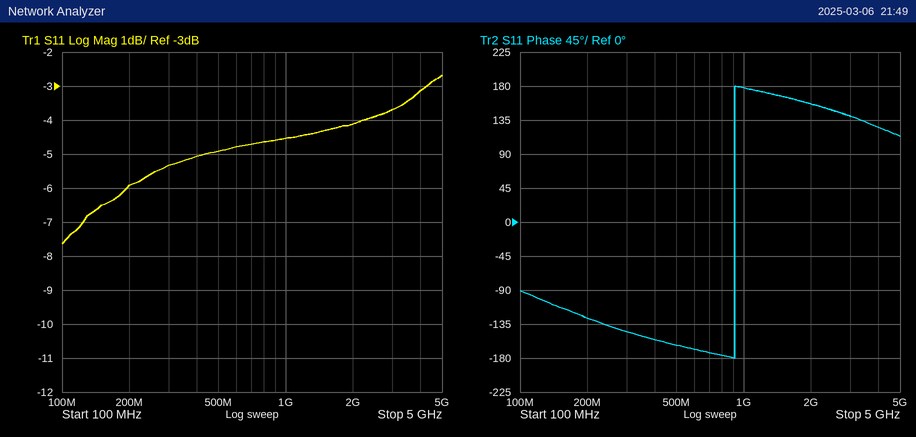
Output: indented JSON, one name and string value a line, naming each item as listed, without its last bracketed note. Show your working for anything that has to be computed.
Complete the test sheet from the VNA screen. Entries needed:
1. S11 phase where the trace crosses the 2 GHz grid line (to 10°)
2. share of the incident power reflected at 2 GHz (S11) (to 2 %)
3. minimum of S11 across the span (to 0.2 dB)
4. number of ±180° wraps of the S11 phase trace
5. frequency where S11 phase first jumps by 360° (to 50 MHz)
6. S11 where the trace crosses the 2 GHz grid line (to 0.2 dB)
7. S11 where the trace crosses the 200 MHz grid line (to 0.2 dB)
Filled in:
{
  "S11 phase where the trace crosses the 2 GHz grid line": "160°",
  "share of the incident power reflected at 2 GHz (S11)": "10^(-4.2/10) ≈ 38 %",
  "minimum of S11 across the span": "-7.6 dB",
  "number of ±180° wraps of the S11 phase trace": "1",
  "frequency where S11 phase first jumps by 360°": "900 MHz",
  "S11 where the trace crosses the 2 GHz grid line": "-4.2 dB",
  "S11 where the trace crosses the 200 MHz grid line": "-6.0 dB"
}
